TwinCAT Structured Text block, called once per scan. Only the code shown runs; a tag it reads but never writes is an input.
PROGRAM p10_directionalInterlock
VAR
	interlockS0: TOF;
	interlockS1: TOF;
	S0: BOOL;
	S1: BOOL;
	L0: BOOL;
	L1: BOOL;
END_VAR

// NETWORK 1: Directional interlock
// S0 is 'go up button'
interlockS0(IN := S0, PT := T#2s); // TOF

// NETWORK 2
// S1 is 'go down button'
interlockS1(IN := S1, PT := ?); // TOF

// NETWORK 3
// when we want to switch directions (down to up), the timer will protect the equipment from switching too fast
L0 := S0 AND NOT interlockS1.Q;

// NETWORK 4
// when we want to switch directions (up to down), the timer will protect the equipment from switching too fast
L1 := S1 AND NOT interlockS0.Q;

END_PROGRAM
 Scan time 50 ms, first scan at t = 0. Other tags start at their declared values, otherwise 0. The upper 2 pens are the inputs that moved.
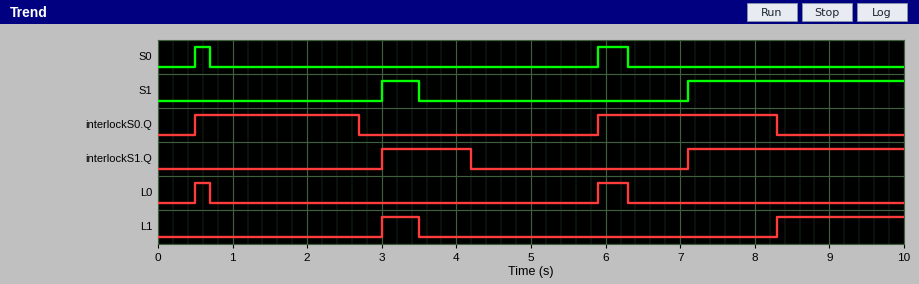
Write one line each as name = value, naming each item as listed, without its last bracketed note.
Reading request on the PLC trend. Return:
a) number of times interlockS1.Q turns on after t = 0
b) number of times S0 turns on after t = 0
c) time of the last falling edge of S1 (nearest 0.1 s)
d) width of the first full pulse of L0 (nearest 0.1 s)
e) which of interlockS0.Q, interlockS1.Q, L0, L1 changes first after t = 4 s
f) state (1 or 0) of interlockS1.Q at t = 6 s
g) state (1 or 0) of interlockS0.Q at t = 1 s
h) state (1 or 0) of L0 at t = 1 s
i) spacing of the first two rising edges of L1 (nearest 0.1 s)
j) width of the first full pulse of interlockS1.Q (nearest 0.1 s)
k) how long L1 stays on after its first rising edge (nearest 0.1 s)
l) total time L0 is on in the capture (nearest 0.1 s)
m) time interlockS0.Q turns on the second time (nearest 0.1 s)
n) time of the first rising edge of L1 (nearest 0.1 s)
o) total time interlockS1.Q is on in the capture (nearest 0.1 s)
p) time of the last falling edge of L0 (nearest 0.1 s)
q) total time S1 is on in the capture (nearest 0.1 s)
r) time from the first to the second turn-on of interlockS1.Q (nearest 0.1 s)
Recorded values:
number of times interlockS1.Q turns on after t = 0 = 2
number of times S0 turns on after t = 0 = 2
time of the last falling edge of S1 = 3.5 s
width of the first full pulse of L0 = 0.2 s
which of interlockS0.Q, interlockS1.Q, L0, L1 changes first after t = 4 s = interlockS1.Q
state (1 or 0) of interlockS1.Q at t = 6 s = 0
state (1 or 0) of interlockS0.Q at t = 1 s = 1
state (1 or 0) of L0 at t = 1 s = 0
spacing of the first two rising edges of L1 = 5.3 s
width of the first full pulse of interlockS1.Q = 1.2 s
how long L1 stays on after its first rising edge = 0.5 s
total time L0 is on in the capture = 0.6 s
time interlockS0.Q turns on the second time = 5.9 s
time of the first rising edge of L1 = 3.0 s
total time interlockS1.Q is on in the capture = 4.1 s
time of the last falling edge of L0 = 6.3 s
total time S1 is on in the capture = 3.4 s
time from the first to the second turn-on of interlockS1.Q = 4.1 s
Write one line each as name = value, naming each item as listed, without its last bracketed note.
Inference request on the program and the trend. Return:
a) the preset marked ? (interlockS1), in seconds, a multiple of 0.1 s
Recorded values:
the preset marked ? (interlockS1), in seconds, a multiple of 0.1 s = 0.7 s
